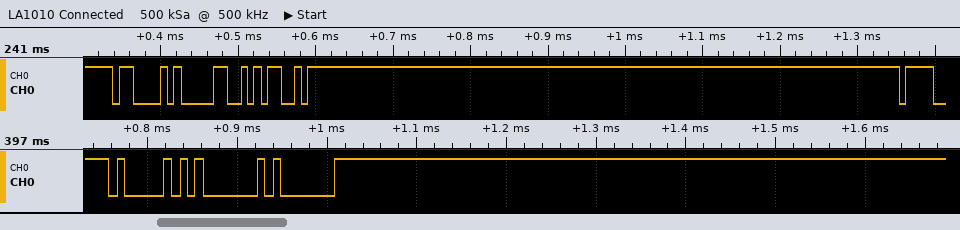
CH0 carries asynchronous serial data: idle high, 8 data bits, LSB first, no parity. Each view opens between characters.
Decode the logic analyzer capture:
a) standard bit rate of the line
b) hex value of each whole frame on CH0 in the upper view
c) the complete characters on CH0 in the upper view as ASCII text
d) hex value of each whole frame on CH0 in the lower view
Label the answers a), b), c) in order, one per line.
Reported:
a) 115200 baud
b) 43, 30, 4D
c) "C0M"
d) 41, 01, 01
